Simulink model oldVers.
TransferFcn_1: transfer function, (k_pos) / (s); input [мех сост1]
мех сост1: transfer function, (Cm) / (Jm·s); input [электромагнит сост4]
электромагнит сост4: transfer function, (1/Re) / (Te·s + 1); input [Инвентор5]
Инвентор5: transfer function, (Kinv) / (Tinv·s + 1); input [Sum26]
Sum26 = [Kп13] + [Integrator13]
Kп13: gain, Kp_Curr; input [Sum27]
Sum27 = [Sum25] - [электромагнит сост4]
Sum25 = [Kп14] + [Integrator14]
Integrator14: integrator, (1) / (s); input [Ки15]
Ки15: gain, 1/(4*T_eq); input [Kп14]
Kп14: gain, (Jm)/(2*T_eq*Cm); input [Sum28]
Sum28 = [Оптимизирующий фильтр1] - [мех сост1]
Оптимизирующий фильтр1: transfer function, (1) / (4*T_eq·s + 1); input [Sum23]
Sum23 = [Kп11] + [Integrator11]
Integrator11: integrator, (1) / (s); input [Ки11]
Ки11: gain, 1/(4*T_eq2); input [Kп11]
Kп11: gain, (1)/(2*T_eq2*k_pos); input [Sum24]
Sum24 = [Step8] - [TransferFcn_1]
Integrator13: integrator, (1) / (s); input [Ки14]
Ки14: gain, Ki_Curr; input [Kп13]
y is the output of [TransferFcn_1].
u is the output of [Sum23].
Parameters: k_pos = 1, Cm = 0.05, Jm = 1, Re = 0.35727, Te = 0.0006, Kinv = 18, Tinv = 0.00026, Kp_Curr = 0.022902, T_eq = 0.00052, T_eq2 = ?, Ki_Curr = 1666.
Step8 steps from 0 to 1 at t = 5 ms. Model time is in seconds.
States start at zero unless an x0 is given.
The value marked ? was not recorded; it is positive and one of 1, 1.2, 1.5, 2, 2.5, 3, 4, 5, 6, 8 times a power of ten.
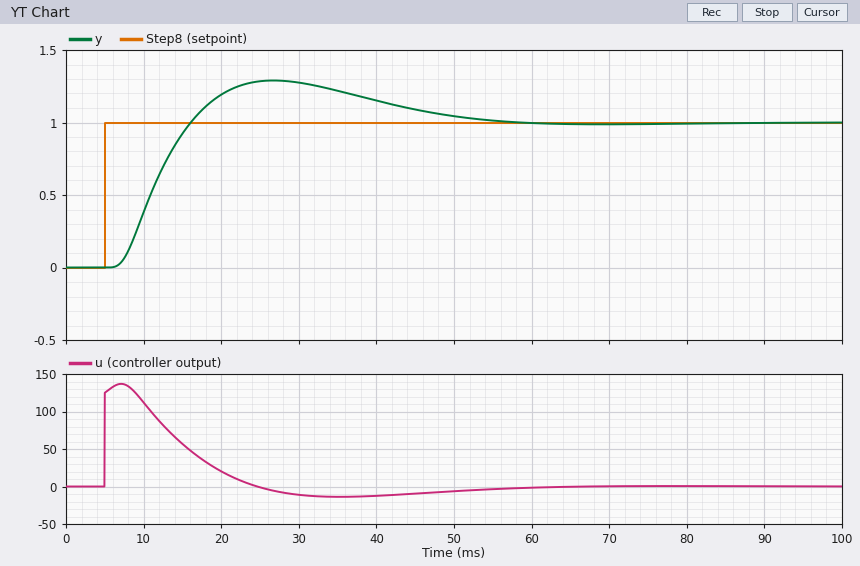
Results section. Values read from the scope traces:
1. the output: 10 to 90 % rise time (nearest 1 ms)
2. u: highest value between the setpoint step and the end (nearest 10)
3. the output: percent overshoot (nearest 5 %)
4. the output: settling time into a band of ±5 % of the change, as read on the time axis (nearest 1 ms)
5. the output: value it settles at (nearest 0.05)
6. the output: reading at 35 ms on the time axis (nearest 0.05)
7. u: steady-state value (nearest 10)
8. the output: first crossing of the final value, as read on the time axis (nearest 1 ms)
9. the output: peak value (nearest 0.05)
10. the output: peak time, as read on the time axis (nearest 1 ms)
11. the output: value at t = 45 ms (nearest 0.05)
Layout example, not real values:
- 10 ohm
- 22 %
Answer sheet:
- 7 ms
- 140
- 30 %
- 49 ms
- 1.00
- 1.20
- 0
- 16 ms
- 1.30
- 27 ms
- 1.10
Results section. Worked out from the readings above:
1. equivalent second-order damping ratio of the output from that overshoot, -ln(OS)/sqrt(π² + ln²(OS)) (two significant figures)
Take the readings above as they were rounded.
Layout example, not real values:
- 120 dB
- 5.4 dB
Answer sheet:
- 0.36
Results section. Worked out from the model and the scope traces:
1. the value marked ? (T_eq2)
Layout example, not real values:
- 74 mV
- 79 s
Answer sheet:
- 0.004
